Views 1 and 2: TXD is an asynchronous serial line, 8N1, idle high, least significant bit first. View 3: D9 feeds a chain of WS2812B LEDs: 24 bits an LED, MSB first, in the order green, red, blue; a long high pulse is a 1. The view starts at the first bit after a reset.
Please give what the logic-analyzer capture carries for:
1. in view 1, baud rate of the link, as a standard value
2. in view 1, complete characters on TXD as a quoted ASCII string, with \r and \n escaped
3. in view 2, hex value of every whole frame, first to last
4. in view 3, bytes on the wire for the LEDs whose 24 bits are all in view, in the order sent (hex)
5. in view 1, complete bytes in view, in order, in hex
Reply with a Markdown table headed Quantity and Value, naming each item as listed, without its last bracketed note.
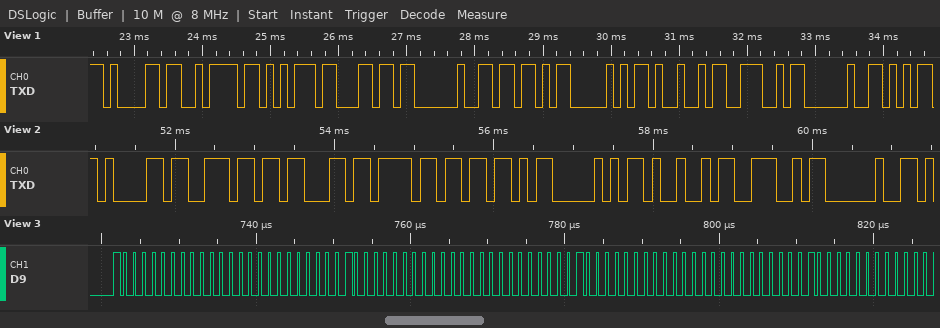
| Quantity | Value |
|---|---|
| in view 1, baud rate of the link, as a standard value | 9600 baud |
| in view 1, complete characters on TXD as a quoted ASCII string, with \r and \n escaped | "azul [PIN " |
| in view 2, hex value of every whole frame, first to last | 0x61 0x6E 0x63 0x6F 0x5B 0x50 0x49 0x4E 0x20 |
| in view 3, bytes on the wire for the LEDs whose 24 bits are all in view, in the order sent | 80 00 00 80 00 00 80 00 00 |
| in view 1, complete bytes in view, in order, in hex | 61 7A 75 6C 20 5B 50 49 4E 20 |
